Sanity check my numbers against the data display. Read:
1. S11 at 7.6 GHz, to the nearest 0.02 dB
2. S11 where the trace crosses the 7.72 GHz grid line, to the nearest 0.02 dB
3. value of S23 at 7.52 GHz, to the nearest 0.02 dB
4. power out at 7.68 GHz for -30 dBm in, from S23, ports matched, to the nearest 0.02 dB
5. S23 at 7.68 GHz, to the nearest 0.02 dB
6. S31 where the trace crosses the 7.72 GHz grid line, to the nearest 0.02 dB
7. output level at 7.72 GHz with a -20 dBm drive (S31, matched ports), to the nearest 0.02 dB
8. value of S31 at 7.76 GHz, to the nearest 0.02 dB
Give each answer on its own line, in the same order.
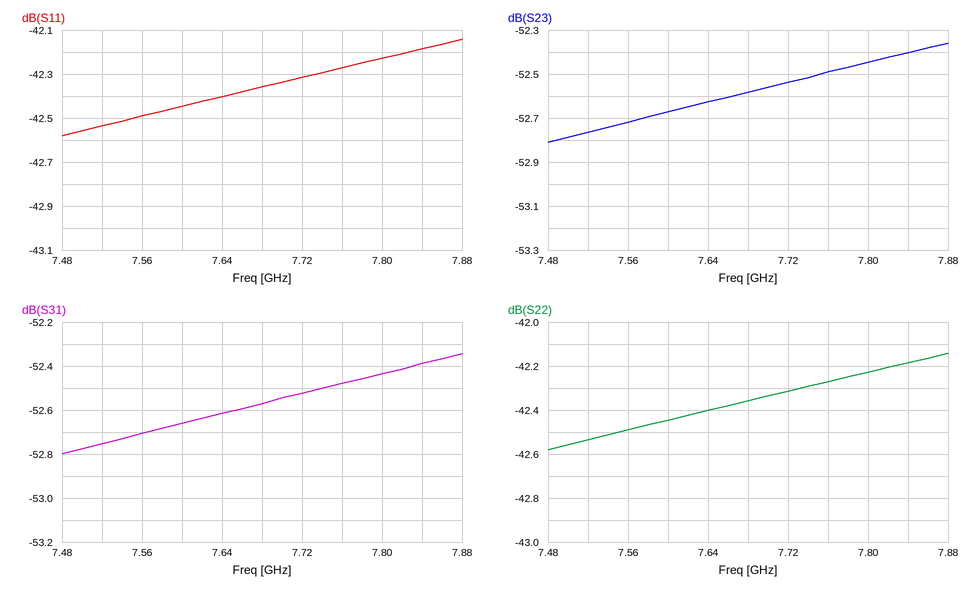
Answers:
-42.44 dB
-42.32 dB
-52.76 dB
-82.58 dBm
-52.58 dB
-52.52 dB
-72.52 dBm
-52.48 dB
